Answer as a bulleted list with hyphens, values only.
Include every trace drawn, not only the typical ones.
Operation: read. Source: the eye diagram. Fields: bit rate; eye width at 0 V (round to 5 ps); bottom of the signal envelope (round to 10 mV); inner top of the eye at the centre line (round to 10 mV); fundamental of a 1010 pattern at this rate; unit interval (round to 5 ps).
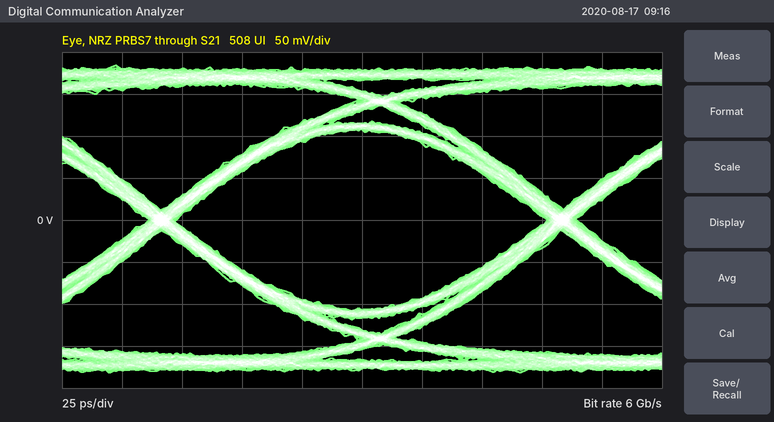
- 6 Gb/s
- 155 ps
- -180 mV
- 110 mV
- 3 GHz
- 165 ps
